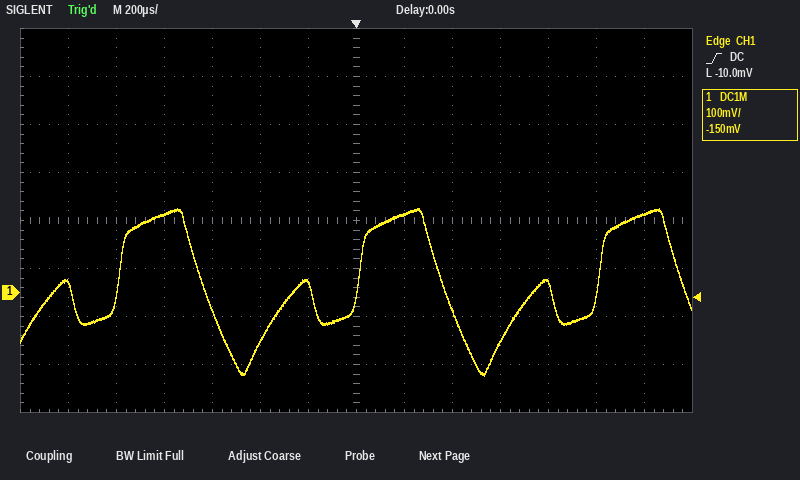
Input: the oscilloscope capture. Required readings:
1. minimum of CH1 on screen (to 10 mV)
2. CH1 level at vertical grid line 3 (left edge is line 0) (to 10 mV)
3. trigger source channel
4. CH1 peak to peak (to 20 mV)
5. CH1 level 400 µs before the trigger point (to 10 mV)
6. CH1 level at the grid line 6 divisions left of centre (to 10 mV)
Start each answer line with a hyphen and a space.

- -170 mV
- 160 mV
- CH1
- 340 mV
- -100 mV
- 20 mV
